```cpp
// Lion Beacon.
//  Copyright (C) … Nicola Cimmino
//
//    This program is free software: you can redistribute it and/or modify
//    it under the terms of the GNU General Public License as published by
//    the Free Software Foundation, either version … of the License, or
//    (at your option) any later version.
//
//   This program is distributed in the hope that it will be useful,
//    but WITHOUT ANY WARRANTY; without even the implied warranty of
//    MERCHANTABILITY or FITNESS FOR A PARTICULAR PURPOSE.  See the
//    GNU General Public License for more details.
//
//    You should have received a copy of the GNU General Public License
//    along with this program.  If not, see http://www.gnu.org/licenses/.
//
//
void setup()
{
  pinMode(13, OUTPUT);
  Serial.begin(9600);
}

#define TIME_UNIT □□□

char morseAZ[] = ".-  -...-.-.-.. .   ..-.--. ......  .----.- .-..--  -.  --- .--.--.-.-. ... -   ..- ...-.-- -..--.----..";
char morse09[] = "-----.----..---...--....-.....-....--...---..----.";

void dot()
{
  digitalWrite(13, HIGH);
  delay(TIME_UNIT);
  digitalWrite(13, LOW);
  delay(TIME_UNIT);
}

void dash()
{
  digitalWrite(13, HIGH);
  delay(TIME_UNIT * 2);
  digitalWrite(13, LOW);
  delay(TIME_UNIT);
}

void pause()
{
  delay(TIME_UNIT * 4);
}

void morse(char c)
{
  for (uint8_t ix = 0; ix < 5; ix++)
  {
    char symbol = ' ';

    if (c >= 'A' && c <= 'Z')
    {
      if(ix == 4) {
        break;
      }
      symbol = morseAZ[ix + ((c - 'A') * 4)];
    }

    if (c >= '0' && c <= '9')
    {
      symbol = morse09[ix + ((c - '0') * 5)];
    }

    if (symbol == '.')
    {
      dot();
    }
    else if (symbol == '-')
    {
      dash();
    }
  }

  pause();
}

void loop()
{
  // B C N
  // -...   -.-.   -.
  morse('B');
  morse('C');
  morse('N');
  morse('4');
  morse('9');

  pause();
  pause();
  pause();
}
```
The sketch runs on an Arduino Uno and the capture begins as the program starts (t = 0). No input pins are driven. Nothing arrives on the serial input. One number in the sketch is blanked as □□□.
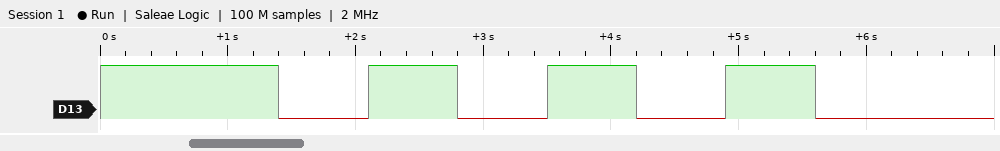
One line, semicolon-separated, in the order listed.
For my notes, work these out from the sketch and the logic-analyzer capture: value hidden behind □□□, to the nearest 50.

700
